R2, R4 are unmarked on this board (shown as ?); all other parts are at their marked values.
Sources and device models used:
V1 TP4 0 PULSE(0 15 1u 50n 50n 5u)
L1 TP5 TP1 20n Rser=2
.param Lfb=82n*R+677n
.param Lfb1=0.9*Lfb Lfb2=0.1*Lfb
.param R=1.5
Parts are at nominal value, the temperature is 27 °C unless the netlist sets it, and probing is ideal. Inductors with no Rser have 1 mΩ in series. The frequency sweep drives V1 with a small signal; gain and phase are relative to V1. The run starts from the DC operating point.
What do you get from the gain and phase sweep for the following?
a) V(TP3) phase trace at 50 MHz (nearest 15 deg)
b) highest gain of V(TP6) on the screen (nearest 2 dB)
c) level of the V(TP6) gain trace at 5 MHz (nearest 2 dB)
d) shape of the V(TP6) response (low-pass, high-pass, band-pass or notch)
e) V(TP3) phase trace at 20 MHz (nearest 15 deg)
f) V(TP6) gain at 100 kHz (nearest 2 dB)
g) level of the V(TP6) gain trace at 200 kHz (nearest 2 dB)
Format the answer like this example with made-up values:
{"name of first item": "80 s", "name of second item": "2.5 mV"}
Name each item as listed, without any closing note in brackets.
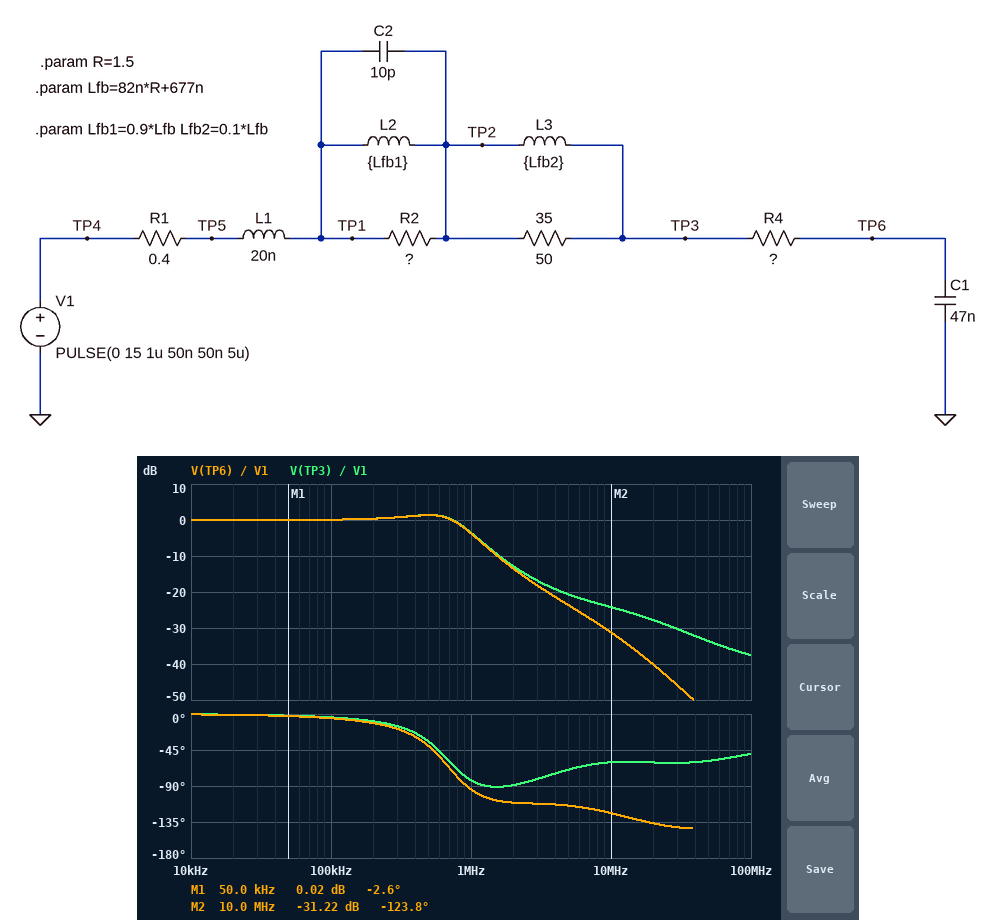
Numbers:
{"V(TP3) phase trace at 50 MHz": "-60 deg", "highest gain of V(TP6) on the screen": "2 dB", "level of the V(TP6) gain trace at 5 MHz": "-24 dB", "shape of the V(TP6) response": "low-pass", "V(TP3) phase trace at 20 MHz": "-60 deg", "V(TP6) gain at 100 kHz": "0 dB", "level of the V(TP6) gain trace at 200 kHz": "0 dB"}
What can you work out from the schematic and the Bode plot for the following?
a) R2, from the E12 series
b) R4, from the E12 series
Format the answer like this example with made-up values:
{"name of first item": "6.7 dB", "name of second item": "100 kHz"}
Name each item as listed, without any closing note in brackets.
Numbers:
{"R2, from the E12 series": "6.8 Ω", "R4, from the E12 series": "0.68 Ω"}
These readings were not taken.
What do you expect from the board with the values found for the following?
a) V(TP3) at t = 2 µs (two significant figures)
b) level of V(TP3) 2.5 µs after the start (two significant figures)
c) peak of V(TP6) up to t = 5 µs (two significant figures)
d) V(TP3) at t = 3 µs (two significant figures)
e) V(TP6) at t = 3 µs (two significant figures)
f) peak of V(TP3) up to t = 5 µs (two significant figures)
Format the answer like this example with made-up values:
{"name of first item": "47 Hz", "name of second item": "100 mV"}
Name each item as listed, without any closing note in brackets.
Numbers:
{"V(TP3) at t = 2 µs": "16 V", "level of V(TP3) 2.5 µs after the start": "15 V", "peak of V(TP6) up to t = 5 µs": "17 V", "V(TP3) at t = 3 µs": "15 V", "V(TP6) at t = 3 µs": "15 V", "peak of V(TP3) up to t = 5 µs": "17 V"}
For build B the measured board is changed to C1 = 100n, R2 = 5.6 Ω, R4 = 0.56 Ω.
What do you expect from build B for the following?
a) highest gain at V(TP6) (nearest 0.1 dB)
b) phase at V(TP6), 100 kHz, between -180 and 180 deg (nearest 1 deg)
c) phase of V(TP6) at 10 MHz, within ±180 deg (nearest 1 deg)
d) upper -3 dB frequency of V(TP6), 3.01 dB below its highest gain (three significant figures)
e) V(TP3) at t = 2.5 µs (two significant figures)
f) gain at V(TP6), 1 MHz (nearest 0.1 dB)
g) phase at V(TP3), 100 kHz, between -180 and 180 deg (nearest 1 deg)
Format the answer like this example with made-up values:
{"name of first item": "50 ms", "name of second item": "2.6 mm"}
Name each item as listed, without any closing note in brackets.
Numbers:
{"highest gain at V(TP6)": "0.5 dB", "phase at V(TP6), 100 kHz, between -180 and 180 deg": "-11 deg", "phase of V(TP6) at 10 MHz, within ±180 deg": "-127 deg", "upper -3 dB frequency of V(TP6), 3.01 dB below its highest gain": "545 kHz", "V(TP3) at t = 2.5 µs": "16 V", "gain at V(TP6), 1 MHz": "-10.7 dB", "phase at V(TP3), 100 kHz, between -180 and 180 deg": "-9 deg"}
